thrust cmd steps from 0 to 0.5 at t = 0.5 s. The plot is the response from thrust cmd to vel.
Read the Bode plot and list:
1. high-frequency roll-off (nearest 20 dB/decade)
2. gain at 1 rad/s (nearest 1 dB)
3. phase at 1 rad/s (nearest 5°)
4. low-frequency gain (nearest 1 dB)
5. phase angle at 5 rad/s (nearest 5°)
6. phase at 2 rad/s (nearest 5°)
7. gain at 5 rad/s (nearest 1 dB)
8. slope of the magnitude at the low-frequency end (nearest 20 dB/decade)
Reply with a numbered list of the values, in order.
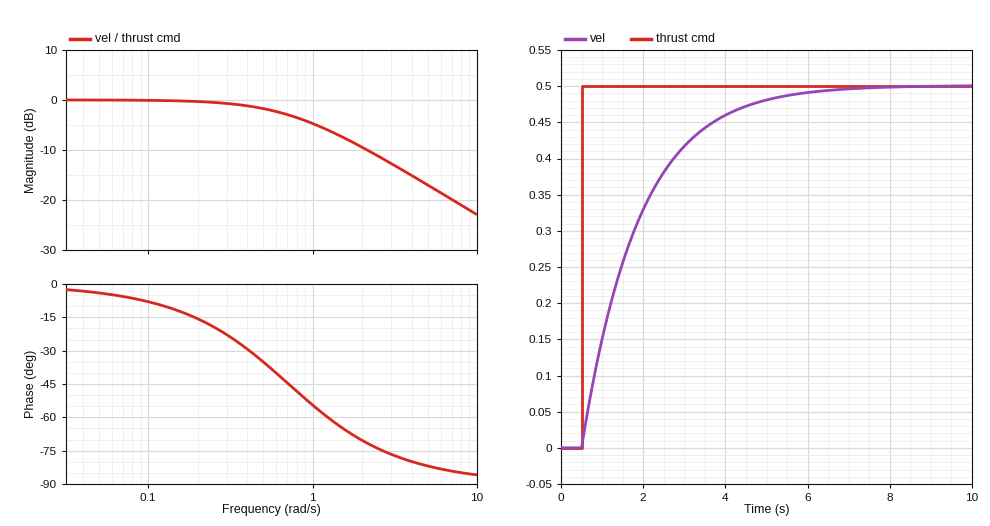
1. -20 dB/decade
2. -5 dB
3. -55°
4. 0 dB
5. -80°
6. -70°
7. -17 dB
8. 0 dB/decade
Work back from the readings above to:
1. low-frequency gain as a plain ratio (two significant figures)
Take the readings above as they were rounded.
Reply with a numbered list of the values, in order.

1. 1.0
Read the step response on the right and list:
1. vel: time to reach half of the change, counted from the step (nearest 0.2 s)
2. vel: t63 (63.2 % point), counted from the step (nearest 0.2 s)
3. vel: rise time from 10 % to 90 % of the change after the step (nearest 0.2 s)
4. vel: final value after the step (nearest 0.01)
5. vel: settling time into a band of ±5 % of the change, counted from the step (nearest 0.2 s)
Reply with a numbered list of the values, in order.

1. 1.0 s
2. 1.4 s
3. 3.0 s
4. 0.50
5. 4.2 s
